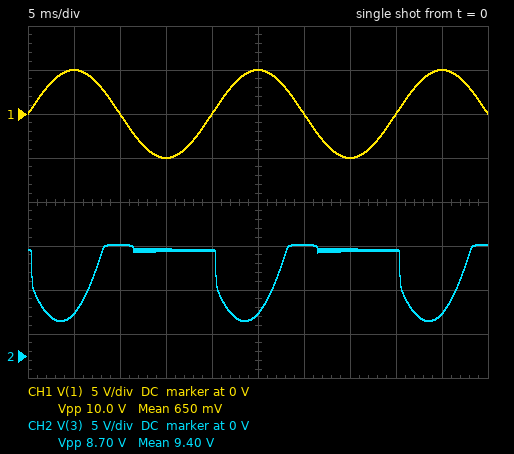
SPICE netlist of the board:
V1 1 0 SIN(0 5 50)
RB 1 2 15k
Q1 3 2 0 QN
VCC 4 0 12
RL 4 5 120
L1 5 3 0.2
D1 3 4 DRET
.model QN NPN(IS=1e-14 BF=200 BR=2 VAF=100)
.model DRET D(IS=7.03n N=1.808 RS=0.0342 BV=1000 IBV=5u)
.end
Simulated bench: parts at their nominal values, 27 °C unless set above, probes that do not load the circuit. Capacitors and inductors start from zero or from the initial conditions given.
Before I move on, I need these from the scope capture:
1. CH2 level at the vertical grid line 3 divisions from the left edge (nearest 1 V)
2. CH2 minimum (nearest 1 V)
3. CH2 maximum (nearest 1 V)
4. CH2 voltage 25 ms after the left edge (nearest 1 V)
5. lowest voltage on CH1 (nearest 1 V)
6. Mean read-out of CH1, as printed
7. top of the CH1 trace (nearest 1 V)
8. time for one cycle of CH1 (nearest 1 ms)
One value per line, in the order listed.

12 V
4 V
13 V
5 V
-5 V
650 mV
5 V
20 ms
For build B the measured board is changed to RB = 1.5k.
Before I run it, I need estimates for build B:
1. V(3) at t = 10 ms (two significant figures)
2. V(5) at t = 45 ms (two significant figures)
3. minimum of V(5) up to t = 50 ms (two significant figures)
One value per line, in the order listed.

13 V
840 mV
180 mV
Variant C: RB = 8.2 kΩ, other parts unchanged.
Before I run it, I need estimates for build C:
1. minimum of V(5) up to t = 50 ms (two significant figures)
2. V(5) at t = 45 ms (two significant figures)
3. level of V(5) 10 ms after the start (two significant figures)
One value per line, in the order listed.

640 mV
1.1 V
10 V
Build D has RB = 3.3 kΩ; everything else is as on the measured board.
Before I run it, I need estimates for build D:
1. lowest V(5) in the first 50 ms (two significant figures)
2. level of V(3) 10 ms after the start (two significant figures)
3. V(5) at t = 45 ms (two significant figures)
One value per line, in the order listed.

230 mV
13 V
870 mV
